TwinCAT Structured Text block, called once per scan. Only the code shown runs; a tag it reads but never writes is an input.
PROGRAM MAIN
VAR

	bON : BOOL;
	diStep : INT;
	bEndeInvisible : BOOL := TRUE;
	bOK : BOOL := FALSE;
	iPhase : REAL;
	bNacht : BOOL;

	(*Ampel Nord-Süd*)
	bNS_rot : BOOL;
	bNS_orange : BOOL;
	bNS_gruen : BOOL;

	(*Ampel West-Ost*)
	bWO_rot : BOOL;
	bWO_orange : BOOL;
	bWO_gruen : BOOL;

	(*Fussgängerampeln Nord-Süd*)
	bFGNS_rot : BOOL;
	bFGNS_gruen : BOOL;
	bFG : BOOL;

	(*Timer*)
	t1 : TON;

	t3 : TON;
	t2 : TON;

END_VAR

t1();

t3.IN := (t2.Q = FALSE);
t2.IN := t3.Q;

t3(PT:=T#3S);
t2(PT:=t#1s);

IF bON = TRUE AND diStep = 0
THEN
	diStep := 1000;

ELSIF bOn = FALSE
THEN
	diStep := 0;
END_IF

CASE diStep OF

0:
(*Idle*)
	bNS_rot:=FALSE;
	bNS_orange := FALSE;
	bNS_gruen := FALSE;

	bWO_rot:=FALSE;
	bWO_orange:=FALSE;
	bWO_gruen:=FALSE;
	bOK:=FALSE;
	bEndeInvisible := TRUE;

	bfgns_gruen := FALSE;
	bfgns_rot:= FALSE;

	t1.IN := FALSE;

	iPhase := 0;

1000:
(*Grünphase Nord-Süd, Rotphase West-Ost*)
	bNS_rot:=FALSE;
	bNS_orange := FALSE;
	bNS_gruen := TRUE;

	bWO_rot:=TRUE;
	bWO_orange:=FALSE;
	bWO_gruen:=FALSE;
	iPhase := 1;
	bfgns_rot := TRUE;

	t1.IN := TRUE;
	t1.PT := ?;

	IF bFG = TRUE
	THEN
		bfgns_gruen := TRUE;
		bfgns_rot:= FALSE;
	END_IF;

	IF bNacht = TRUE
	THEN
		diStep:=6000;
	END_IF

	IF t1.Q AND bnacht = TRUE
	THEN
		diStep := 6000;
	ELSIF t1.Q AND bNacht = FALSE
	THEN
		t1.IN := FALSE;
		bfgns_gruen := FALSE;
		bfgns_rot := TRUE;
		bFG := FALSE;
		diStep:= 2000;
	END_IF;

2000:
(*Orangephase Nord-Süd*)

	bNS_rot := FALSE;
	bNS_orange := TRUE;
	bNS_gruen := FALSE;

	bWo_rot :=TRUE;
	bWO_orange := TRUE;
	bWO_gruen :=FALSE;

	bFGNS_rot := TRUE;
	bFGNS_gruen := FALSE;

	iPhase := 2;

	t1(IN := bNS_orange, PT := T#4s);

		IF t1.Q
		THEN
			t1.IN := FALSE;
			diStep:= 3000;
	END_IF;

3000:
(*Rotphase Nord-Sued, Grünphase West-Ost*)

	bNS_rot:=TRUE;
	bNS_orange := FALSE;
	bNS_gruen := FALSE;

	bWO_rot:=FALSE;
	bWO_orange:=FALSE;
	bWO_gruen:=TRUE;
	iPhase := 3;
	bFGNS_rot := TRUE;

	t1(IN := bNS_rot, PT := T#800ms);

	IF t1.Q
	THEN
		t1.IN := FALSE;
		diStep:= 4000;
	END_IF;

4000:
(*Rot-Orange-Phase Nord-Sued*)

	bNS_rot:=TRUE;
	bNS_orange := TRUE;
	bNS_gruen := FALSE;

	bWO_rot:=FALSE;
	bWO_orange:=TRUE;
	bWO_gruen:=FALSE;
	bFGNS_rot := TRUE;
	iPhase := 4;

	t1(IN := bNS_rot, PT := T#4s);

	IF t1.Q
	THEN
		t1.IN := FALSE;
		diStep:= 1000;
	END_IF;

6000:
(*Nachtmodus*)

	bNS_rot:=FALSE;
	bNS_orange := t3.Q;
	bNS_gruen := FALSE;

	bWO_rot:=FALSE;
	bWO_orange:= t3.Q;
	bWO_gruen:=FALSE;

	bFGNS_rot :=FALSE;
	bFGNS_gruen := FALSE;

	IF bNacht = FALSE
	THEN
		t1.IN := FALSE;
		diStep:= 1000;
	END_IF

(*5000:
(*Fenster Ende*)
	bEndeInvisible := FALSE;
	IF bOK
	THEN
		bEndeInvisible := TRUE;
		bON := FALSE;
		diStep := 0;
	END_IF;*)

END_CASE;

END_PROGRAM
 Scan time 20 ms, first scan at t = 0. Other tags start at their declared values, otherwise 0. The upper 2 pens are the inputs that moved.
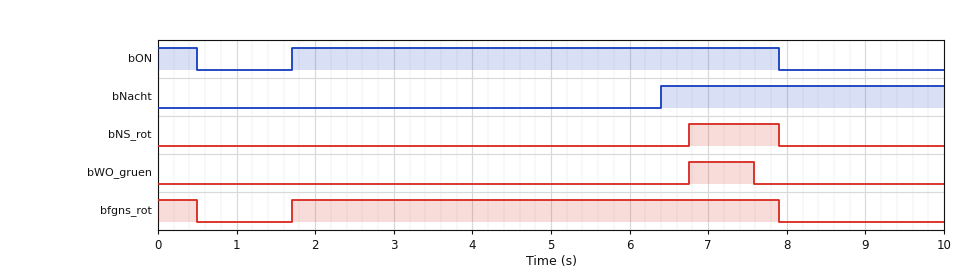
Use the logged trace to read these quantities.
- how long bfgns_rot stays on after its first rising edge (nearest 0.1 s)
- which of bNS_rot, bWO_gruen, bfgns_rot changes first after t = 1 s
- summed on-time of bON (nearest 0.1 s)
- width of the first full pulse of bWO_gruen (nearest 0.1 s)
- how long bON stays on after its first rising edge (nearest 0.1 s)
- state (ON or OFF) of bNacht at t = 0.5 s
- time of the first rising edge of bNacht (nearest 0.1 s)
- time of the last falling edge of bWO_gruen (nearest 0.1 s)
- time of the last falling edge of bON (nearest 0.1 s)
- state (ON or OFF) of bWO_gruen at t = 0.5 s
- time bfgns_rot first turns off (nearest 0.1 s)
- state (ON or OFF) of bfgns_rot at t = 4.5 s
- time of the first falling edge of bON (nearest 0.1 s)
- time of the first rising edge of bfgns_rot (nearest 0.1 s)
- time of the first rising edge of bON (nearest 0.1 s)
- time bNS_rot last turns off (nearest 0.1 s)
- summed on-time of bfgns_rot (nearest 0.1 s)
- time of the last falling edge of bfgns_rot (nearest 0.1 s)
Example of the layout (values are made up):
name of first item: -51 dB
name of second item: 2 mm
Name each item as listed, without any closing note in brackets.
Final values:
how long bfgns_rot stays on after its first rising edge: 6.2 s
which of bNS_rot, bWO_gruen, bfgns_rot changes first after t = 1 s: bfgns_rot
summed on-time of bON: 6.7 s
width of the first full pulse of bWO_gruen: 0.8 s
how long bON stays on after its first rising edge: 6.2 s
state (ON or OFF) of bNacht at t = 0.5 s: OFF
time of the first rising edge of bNacht: 6.4 s
time of the last falling edge of bWO_gruen: 7.6 s
time of the last falling edge of bON: 7.9 s
state (ON or OFF) of bWO_gruen at t = 0.5 s: OFF
time bfgns_rot first turns off: 0.5 s
state (ON or OFF) of bfgns_rot at t = 4.5 s: ON
time of the first falling edge of bON: 0.5 s
time of the first rising edge of bfgns_rot: 1.7 s
time of the first rising edge of bON: 1.7 s
time bNS_rot last turns off: 7.9 s
summed on-time of bfgns_rot: 6.7 s
time of the last falling edge of bfgns_rot: 7.9 s
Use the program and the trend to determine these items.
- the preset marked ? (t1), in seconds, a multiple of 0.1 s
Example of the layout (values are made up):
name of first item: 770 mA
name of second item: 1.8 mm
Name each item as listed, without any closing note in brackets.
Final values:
the preset marked ? (t1), in seconds, a multiple of 0.1 s: 1.0 s
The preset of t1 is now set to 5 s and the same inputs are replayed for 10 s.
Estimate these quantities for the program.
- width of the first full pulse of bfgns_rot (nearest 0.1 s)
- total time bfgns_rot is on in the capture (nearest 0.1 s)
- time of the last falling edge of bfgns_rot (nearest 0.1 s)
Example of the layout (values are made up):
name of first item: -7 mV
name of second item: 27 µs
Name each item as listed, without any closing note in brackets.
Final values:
width of the first full pulse of bfgns_rot: 4.7 s
total time bfgns_rot is on in the capture: 5.2 s
time of the last falling edge of bfgns_rot: 6.4 s
